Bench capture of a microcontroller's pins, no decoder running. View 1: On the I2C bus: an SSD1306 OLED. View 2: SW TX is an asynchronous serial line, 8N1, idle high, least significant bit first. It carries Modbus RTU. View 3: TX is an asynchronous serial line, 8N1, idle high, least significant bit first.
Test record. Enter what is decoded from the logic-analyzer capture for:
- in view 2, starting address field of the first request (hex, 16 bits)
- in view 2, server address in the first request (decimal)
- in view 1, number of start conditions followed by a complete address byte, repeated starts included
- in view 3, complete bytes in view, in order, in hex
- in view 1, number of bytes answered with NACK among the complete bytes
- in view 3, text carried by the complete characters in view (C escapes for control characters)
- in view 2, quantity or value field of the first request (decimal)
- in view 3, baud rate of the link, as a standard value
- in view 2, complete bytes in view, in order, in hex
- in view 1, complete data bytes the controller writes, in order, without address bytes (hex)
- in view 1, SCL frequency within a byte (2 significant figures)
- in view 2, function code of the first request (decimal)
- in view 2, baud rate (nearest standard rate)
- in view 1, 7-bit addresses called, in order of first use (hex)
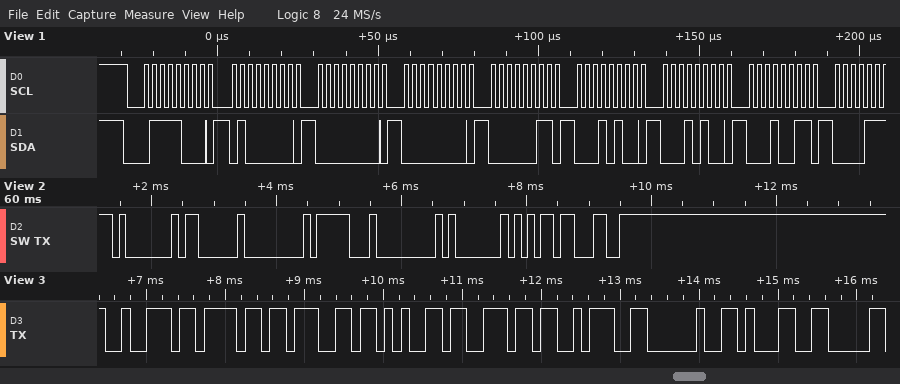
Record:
0x001F
1
1
72 6F 67 65 6E 3A 20 31
0
"rogen: 1"
1
9600 baud
0x01 0x03 0x00 0x1F 0x00 0x01 0xB5 0xCC
40 00 00 03 14 14 13
400 kHz
3
9600 baud
0x3C
